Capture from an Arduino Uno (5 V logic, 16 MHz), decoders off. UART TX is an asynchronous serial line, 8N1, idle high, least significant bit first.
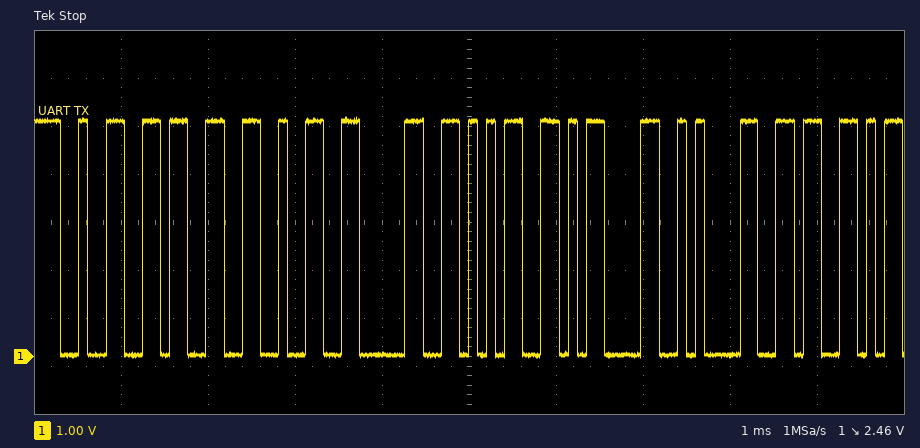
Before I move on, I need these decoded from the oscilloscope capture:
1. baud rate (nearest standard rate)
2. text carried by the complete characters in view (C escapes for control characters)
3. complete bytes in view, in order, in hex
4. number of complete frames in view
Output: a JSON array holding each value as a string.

["9600 baud", "\"23205\\r\\n6\"", "0x32 0x33 0x32 0x30 0x35 0x0D 0x0A 0x36", "8"]
